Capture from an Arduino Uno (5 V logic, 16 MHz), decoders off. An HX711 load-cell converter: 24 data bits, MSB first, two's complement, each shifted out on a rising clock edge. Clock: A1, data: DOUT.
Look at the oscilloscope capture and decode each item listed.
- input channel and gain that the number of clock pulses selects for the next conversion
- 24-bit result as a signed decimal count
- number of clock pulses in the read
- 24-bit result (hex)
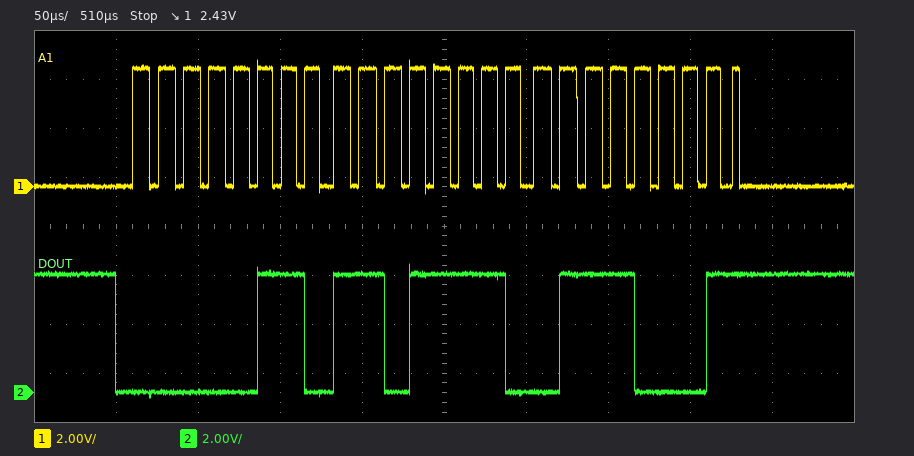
channel A, gain 128
450161
25
0x06DE71
